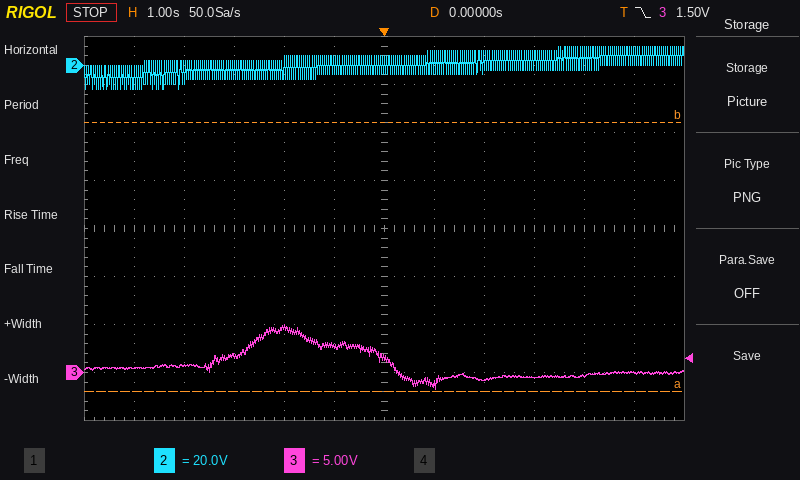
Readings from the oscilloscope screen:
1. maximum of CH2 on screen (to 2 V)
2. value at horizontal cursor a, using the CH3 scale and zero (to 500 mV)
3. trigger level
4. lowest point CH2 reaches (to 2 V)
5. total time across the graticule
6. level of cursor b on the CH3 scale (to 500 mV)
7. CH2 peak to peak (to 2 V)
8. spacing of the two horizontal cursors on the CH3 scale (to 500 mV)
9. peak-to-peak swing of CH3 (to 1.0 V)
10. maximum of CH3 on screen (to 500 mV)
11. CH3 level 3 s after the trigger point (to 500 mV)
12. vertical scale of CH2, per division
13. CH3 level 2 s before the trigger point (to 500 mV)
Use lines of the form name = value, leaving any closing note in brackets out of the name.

maximum of CH2 on screen = 8 V
value at horizontal cursor a, using the CH3 scale and zero = -2.0 V
trigger level = 1.50 V
lowest point CH2 reaches = -10 V
total time across the graticule = 12 s
level of cursor b on the CH3 scale = 26.0 V
CH2 peak to peak = 18 V
spacing of the two horizontal cursors on the CH3 scale = 28.0 V
peak-to-peak swing of CH3 = 7.0 V
maximum of CH3 on screen = 5.0 V
CH3 level 3 s after the trigger point = -500 mV
vertical scale of CH2, per division = 20 V
CH3 level 2 s before the trigger point = 4.5 V
